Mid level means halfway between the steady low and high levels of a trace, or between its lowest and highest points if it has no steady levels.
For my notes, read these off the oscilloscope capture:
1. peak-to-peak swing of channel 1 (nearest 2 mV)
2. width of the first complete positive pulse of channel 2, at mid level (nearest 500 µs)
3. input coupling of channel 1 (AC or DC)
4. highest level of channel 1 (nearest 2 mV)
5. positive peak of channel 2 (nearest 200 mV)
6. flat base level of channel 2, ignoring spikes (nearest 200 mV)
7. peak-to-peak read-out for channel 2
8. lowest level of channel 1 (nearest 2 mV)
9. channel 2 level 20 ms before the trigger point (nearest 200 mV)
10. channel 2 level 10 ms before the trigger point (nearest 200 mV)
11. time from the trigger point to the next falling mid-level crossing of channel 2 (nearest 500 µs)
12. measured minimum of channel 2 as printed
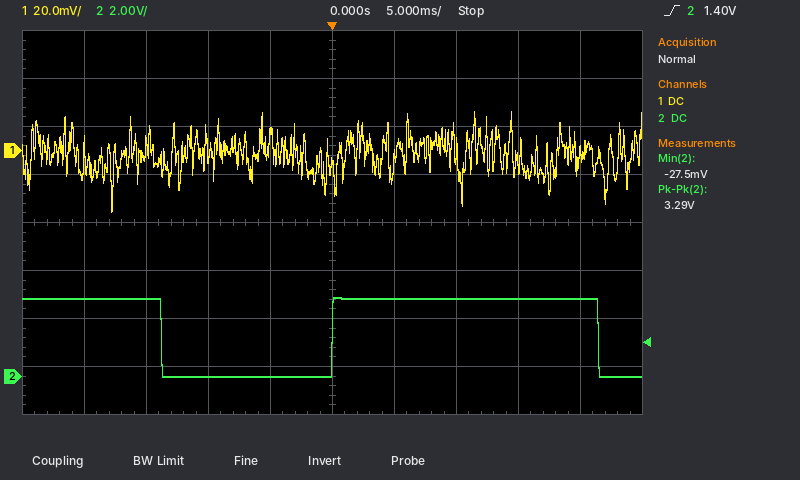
42 mV
21.5 ms
DC
16 mV
3.2 V
0.0 V
3.29 V
-26 mV
3.2 V
0.0 V
21.5 ms
-27.5 mV
